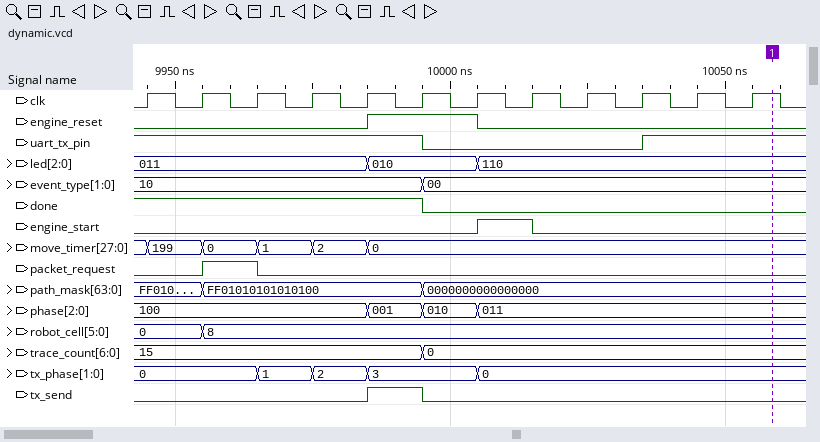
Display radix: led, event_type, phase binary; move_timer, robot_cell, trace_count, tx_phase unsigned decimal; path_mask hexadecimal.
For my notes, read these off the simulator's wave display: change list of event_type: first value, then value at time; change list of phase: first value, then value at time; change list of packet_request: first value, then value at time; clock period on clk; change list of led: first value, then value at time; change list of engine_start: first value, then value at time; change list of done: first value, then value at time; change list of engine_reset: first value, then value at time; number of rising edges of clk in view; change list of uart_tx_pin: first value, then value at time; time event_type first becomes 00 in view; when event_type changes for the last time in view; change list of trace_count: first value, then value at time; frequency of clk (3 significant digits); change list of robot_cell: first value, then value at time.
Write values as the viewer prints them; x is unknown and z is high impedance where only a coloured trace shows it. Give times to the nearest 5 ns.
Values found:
10, 00 at 9995 ns
100, 001 at 9985 ns, 010 at 9995 ns, 011 at 10005 ns
0, 1 at 9955 ns, 0 at 9965 ns
10 ns
011, 010 at 9985 ns, 110 at 10005 ns
0, 1 at 10005 ns, 0 at 10015 ns
1, 0 at 9995 ns
0, 1 at 9985 ns, 0 at 10005 ns
12
1, 0 at 9995 ns, 1 at 10035 ns
9995 ns
9995 ns
15, 0 at 9995 ns
100 MHz
0, 8 at 9955 ns
